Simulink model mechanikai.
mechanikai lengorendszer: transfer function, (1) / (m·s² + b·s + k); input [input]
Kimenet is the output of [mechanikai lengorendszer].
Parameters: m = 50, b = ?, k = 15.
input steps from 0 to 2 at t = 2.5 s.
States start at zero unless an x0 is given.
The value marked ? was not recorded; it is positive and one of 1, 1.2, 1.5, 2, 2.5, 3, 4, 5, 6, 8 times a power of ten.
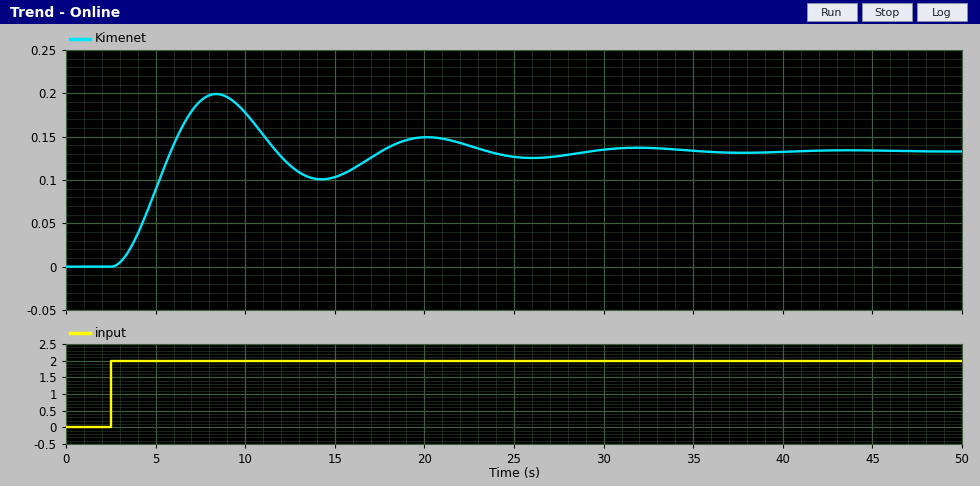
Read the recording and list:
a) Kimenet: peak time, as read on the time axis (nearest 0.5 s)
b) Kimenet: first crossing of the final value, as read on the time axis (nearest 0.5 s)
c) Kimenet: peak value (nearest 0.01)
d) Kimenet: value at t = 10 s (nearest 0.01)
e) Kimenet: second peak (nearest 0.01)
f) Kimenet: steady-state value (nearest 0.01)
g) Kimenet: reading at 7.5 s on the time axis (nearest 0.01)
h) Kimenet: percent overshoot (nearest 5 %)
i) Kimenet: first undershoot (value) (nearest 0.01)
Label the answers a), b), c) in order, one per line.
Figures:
a) 8.5 s
b) 6.0 s
c) 0.20
d) 0.18
e) 0.15
f) 0.13
g) 0.19
h) 50 %
i) 0.10
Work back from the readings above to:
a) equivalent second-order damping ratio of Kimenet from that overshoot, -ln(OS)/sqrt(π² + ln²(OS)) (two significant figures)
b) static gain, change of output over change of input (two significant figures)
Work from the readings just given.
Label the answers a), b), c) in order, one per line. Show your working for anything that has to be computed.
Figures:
a) ln(0.5) = -0.693; 0.693 / sqrt(9.870 + 0.480) = 0.22
b) (0.13 - 0) / (2 - 0) = 0.065
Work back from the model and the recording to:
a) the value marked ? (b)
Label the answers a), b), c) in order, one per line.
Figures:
a) 12
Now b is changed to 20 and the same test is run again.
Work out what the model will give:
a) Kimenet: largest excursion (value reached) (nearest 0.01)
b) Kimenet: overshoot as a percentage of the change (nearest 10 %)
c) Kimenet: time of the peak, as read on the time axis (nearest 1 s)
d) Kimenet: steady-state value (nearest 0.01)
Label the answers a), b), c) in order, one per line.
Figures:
a) 0.17
b) 30 %
c) 9 s
d) 0.13
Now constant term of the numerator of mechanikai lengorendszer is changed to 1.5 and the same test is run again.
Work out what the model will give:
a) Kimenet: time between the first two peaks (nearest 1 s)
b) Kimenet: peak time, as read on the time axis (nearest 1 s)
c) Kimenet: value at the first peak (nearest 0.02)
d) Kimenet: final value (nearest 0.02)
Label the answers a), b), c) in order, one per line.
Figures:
a) 12 s
b) 8 s
c) 0.30
d) 0.20
